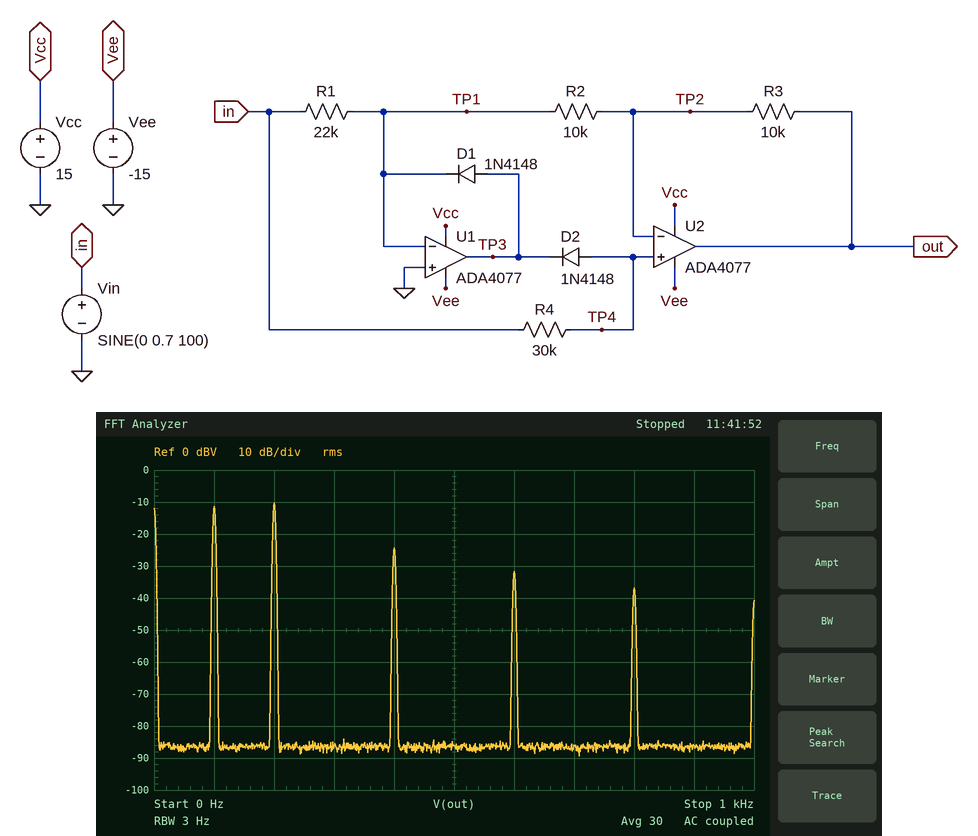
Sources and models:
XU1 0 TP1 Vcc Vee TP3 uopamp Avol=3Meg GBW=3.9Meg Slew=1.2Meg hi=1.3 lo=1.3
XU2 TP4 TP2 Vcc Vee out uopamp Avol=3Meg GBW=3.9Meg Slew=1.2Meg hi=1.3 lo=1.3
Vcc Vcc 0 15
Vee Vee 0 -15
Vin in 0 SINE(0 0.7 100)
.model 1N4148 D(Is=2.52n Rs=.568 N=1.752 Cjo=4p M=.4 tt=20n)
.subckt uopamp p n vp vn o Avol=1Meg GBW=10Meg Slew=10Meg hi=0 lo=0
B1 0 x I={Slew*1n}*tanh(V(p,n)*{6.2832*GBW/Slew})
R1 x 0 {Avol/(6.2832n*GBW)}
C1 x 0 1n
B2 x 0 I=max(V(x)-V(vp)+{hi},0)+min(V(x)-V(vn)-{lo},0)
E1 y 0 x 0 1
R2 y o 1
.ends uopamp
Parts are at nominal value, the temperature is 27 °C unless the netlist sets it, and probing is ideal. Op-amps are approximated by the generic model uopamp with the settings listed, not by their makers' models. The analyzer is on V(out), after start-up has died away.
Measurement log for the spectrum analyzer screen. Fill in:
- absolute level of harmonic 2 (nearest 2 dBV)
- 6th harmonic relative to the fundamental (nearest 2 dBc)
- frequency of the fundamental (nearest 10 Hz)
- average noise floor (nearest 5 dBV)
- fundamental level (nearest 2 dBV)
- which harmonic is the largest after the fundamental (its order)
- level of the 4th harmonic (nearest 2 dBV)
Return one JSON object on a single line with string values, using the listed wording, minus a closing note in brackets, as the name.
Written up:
{"absolute level of harmonic 2": "-10 dBV", "6th harmonic relative to the fundamental": "-20 dBc", "frequency of the fundamental": "100 Hz", "average noise floor": "-85 dBV", "fundamental level": "-12 dBV", "which harmonic is the largest after the fundamental": "2", "level of the 4th harmonic": "-24 dBV"}
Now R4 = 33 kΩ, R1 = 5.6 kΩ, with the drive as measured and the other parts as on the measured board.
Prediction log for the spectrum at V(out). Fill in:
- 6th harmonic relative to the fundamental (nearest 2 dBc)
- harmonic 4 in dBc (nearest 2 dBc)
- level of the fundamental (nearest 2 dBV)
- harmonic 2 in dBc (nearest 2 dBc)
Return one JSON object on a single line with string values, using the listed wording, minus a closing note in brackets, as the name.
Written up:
{"6th harmonic relative to the fundamental": "-18 dBc", "harmonic 4 in dBc": "-10 dBc", "level of the fundamental": "-8 dBV", "harmonic 2 in dBc": "4 dBc"}
